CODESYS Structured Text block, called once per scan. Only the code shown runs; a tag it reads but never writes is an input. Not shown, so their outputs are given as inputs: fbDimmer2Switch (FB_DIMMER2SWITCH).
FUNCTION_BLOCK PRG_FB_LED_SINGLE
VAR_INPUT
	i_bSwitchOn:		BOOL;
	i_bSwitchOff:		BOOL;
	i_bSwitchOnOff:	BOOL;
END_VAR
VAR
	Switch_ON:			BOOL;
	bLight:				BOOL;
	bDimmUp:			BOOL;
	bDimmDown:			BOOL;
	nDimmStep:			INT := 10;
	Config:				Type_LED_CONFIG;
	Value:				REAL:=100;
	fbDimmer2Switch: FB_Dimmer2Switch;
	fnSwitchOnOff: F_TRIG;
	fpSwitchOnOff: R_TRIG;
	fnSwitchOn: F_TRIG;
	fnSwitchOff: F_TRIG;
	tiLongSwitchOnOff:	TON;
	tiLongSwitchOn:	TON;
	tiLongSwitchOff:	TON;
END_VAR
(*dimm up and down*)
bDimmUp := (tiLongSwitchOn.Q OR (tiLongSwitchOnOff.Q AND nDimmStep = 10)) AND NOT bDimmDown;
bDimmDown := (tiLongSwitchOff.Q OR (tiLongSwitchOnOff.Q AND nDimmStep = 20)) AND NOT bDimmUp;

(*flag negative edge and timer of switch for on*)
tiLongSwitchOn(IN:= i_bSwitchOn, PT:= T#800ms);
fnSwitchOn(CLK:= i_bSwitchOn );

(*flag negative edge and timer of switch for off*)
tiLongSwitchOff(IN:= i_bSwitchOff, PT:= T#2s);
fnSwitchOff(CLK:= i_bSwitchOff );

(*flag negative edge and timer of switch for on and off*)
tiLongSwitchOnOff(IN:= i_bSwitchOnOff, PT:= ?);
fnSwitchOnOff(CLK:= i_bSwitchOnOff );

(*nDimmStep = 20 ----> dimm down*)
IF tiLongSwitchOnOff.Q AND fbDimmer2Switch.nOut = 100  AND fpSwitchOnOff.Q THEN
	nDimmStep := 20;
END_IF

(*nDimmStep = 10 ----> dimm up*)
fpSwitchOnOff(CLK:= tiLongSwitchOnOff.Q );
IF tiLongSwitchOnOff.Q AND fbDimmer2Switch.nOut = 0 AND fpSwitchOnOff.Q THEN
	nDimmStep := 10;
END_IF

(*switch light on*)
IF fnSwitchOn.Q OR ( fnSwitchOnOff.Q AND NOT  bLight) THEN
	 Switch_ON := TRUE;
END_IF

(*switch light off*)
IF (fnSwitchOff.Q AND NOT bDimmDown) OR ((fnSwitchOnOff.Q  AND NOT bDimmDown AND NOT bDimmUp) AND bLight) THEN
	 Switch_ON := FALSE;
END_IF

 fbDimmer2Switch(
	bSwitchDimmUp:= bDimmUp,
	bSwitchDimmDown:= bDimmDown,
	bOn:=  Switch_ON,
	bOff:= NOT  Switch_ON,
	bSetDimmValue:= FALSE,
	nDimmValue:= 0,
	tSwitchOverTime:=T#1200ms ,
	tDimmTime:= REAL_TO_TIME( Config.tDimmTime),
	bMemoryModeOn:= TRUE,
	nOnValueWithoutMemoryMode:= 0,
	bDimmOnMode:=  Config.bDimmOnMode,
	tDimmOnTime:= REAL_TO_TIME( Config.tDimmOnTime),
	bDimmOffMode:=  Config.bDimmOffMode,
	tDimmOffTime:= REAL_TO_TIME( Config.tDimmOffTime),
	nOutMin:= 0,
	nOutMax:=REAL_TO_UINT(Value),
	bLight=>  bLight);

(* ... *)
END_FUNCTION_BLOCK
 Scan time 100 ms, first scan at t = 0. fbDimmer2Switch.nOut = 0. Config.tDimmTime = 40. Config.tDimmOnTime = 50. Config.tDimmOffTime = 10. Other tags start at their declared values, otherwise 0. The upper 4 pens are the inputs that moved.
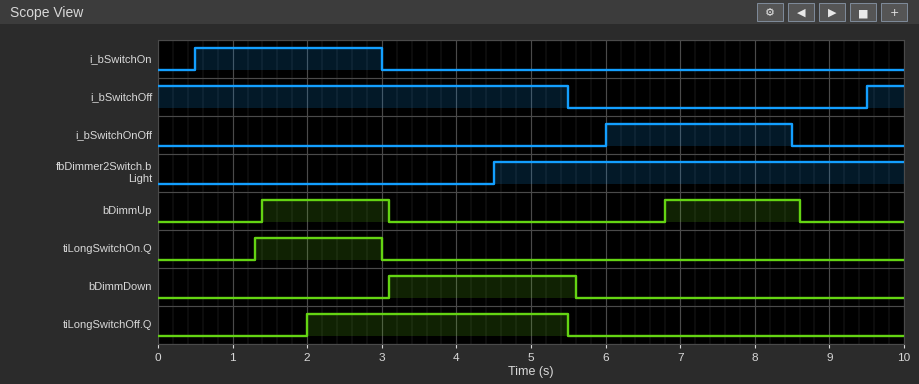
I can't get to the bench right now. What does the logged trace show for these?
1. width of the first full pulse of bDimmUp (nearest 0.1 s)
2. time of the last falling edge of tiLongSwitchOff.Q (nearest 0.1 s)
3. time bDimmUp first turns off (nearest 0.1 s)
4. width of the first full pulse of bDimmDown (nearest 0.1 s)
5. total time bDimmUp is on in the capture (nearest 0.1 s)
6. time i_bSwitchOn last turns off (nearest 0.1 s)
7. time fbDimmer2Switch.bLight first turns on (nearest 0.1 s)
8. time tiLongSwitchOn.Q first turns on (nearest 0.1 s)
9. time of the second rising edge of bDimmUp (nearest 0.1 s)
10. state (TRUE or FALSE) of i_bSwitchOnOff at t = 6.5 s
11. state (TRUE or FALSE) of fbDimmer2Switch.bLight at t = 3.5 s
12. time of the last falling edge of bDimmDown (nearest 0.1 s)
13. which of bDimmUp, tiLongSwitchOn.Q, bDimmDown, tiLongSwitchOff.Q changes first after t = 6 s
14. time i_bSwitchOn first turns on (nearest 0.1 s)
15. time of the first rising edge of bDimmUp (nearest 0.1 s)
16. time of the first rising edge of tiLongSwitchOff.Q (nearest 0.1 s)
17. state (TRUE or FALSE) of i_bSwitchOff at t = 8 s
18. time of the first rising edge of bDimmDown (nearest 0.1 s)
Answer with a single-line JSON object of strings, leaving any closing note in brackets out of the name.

{"width of the first full pulse of bDimmUp": "1.7 s", "time of the last falling edge of tiLongSwitchOff.Q": "5.5 s", "time bDimmUp first turns off": "3.1 s", "width of the first full pulse of bDimmDown": "2.5 s", "total time bDimmUp is on in the capture": "3.5 s", "time i_bSwitchOn last turns off": "3.0 s", "time fbDimmer2Switch.bLight first turns on": "4.5 s", "time tiLongSwitchOn.Q first turns on": "1.3 s", "time of the second rising edge of bDimmUp": "6.8 s", "state (TRUE or FALSE) of i_bSwitchOnOff at t = 6.5 s": "TRUE", "state (TRUE or FALSE) of fbDimmer2Switch.bLight at t = 3.5 s": "FALSE", "time of the last falling edge of bDimmDown": "5.6 s", "which of bDimmUp, tiLongSwitchOn.Q, bDimmDown, tiLongSwitchOff.Q changes first after t = 6 s": "bDimmUp", "time i_bSwitchOn first turns on": "0.5 s", "time of the first rising edge of bDimmUp": "1.4 s", "time of the first rising edge of tiLongSwitchOff.Q": "2.0 s", "state (TRUE or FALSE) of i_bSwitchOff at t = 8 s": "FALSE", "time of the first rising edge of bDimmDown": "3.1 s"}
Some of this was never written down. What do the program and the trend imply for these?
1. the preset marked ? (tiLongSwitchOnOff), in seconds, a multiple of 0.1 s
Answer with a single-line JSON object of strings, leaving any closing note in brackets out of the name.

{"the preset marked ? (tiLongSwitchOnOff), in seconds, a multiple of 0.1 s": "0.7 s"}
